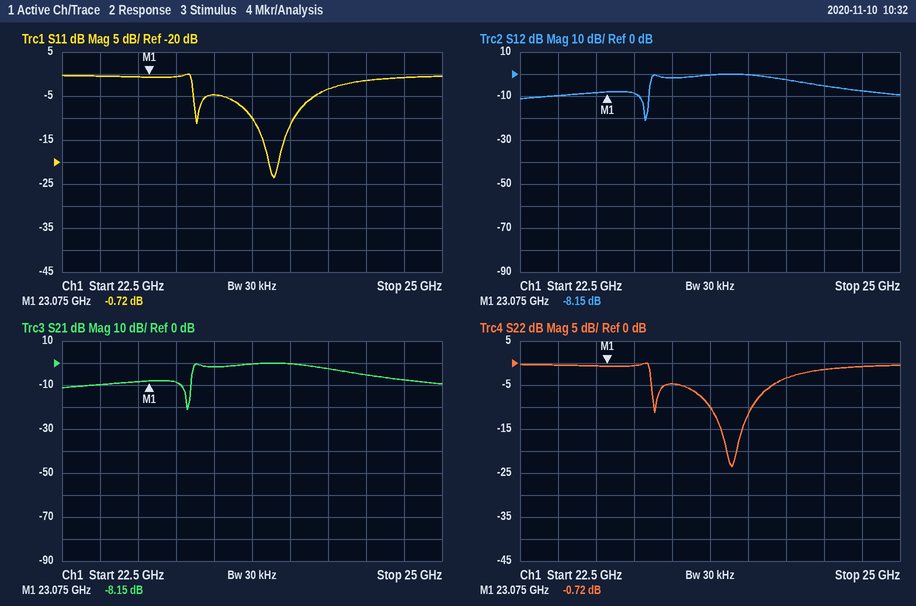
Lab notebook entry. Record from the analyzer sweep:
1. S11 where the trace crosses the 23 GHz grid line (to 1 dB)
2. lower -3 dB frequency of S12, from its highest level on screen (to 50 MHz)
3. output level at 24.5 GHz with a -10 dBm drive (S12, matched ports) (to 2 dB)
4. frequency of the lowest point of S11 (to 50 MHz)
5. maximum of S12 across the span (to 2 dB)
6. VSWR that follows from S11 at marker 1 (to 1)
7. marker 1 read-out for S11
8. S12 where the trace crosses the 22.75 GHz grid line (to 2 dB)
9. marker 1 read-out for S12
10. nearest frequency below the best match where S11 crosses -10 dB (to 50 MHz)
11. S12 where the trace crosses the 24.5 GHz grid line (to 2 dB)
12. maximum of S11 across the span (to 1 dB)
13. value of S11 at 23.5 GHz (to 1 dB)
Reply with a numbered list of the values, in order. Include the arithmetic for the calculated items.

1. -1 dB
2. 23.35 GHz
3. -10 dBm + (-6 dB) = -16 dBm
4. 23.90 GHz
5. 0 dB
6. (1 + 0.9204)/(1 − 0.9204) ≈ 24
7. -0.72 dB
8. -10 dB
9. -8.15 dB
10. 23.75 GHz
11. -6 dB
12. 0 dB
13. -5 dB
